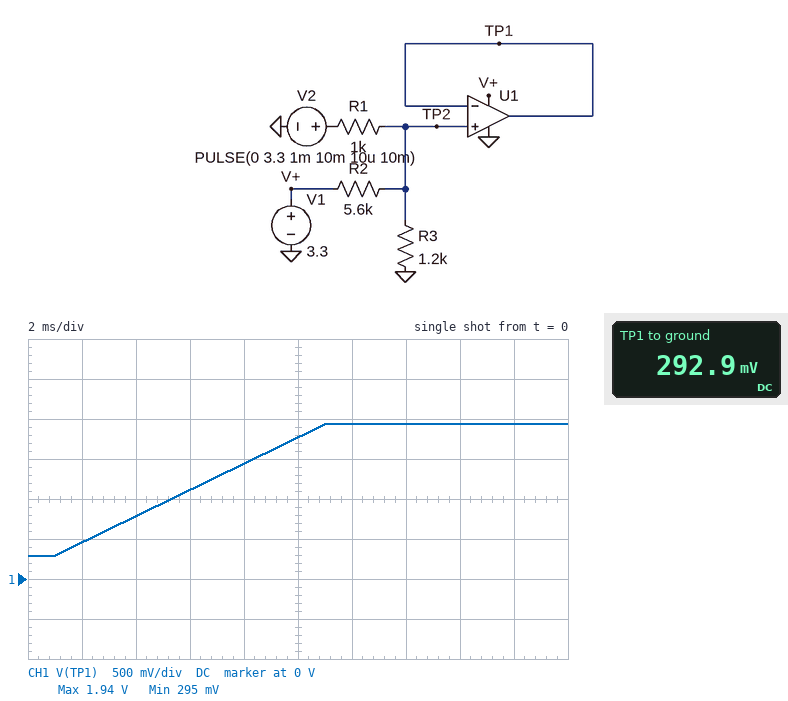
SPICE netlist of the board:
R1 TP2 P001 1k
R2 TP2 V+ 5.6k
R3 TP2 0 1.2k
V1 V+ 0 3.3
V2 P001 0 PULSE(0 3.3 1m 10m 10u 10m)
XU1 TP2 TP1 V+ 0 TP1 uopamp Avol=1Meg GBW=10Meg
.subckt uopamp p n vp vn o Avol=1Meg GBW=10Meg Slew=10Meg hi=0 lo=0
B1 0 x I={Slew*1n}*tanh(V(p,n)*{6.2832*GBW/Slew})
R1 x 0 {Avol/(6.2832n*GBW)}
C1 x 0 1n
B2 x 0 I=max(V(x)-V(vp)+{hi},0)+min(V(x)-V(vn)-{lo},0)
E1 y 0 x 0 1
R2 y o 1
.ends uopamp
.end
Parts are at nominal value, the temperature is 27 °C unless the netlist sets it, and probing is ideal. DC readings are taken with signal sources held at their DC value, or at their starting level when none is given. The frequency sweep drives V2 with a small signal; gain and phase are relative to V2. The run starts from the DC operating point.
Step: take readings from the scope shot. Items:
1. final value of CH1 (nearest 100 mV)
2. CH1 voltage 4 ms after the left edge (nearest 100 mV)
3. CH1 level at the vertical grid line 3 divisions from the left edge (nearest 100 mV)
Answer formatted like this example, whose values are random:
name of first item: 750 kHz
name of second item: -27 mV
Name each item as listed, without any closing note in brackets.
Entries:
final value of CH1: 1.9 V
CH1 voltage 4 ms after the left edge: 800 mV
CH1 level at the vertical grid line 3 divisions from the left edge: 1.1 V
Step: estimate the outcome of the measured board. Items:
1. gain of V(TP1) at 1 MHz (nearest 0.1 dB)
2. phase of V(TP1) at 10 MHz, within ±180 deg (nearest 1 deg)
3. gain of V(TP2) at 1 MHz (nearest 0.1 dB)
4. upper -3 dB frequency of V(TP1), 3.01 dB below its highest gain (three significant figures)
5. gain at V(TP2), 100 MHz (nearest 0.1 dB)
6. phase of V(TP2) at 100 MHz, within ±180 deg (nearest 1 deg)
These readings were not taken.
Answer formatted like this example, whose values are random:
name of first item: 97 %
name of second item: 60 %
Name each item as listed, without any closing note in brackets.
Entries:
gain of V(TP1) at 1 MHz: -6.1 dB
phase of V(TP1) at 10 MHz, within ±180 deg: -45 deg
gain of V(TP2) at 1 MHz: -6.1 dB
upper -3 dB frequency of V(TP1), 3.01 dB below its highest gain: 10.0 MHz
gain at V(TP2), 100 MHz: -6.1 dB
phase of V(TP2) at 100 MHz, within ±180 deg: 0 deg
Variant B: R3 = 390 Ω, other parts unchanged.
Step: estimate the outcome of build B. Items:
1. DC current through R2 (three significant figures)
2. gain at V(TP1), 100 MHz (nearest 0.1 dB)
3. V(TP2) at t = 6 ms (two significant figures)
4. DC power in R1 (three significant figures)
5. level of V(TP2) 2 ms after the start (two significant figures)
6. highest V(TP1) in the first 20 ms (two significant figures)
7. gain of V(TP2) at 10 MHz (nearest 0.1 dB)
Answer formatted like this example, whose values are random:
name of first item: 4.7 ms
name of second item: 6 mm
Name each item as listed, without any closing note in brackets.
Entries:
DC current through R2: 561 µA
gain at V(TP1), 100 MHz: -31.5 dB
V(TP2) at t = 6 ms: 600 mV
DC power in R1: 24.8 µW
level of V(TP2) 2 ms after the start: 250 mV
highest V(TP1) in the first 20 ms: 1.0 V
gain of V(TP2) at 10 MHz: -11.5 dB
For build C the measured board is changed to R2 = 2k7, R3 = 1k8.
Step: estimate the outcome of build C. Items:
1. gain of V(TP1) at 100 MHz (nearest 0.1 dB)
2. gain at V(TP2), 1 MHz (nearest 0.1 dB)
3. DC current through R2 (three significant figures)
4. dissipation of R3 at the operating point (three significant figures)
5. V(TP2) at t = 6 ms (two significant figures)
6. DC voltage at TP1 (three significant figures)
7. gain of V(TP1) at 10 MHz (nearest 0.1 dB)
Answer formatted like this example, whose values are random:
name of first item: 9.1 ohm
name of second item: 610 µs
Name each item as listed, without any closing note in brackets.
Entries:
gain of V(TP1) at 100 MHz: -25.7 dB
gain at V(TP2), 1 MHz: -5.7 dB
DC current through R2: 987 µA
dissipation of R3 at the operating point: 224 µW
V(TP2) at t = 6 ms: 1.5 V
DC voltage at TP1: 635 mV
gain of V(TP1) at 10 MHz: -8.7 dB
